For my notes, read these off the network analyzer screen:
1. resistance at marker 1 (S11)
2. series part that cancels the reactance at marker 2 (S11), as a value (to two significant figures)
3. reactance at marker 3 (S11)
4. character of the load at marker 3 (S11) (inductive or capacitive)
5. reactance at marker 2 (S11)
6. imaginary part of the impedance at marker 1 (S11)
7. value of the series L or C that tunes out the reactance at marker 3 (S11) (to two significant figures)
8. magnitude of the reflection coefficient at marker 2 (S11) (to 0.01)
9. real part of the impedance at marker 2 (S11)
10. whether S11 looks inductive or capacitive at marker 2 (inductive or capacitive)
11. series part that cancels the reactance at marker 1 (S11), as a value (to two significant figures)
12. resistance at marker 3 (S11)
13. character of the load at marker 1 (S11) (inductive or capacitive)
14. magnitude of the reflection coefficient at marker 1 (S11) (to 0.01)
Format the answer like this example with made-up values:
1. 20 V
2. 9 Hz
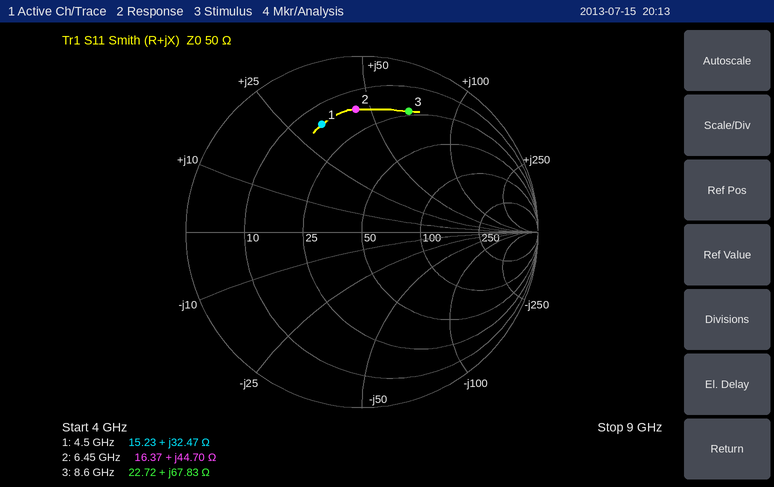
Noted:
1. 15.23 Ω
2. 550 fF
3. +67.83 Ω
4. inductive
5. +44.70 Ω
6. +32.47 Ω
7. 270 fF
8. 0.70
9. 16.37 Ω
10. inductive
11. 1.1 pF
12. 22.72 Ω
13. inductive
14. 0.65
